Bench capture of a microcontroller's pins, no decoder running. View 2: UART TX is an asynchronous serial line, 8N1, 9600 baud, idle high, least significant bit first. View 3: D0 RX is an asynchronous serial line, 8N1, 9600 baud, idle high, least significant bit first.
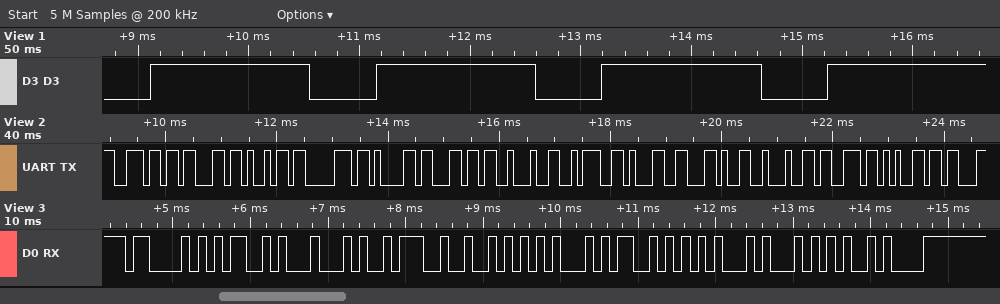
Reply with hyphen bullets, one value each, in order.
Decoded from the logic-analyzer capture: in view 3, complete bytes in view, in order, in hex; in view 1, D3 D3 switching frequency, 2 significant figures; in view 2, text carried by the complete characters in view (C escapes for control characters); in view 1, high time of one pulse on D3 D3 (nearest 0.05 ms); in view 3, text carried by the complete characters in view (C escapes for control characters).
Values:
- 43 4D 44 3A 52 45 53 45 54 0A
- 490 Hz
- "ncipal\":1,\"se"
- 1.45 ms
- "CMD:RESET\n"
